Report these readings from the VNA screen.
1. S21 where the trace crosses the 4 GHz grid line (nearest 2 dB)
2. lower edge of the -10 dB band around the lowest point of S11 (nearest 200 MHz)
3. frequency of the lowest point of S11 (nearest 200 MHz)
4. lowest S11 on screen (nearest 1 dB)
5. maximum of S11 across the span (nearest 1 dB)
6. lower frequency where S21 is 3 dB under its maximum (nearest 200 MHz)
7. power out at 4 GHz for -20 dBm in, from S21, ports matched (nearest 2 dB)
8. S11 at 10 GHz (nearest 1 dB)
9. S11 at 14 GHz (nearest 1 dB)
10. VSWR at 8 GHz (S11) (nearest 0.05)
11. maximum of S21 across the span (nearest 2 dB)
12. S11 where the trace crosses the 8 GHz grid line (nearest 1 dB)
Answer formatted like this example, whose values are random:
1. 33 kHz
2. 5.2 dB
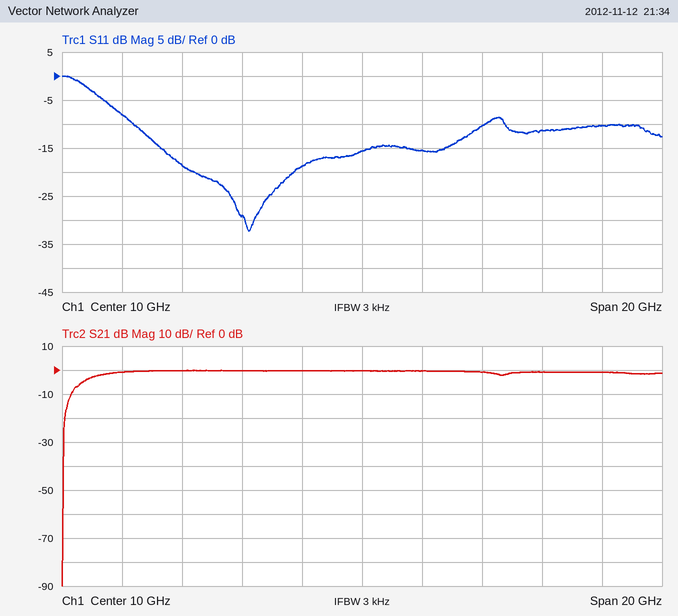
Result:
1. 0 dB
2. 2.4 GHz
3. 6.2 GHz
4. -32 dB
5. 0 dB
6. 1.0 GHz
7. -20 dBm
8. -16 dB
9. -10 dB
10. 1.25
11. 0 dB
12. -19 dB
